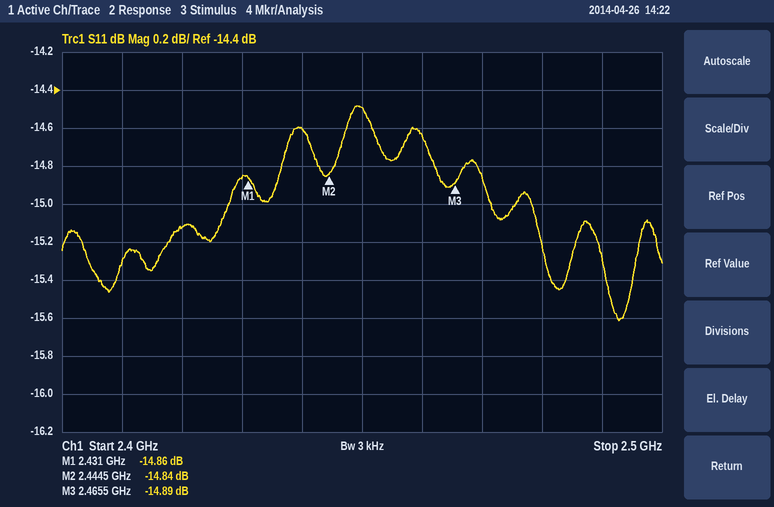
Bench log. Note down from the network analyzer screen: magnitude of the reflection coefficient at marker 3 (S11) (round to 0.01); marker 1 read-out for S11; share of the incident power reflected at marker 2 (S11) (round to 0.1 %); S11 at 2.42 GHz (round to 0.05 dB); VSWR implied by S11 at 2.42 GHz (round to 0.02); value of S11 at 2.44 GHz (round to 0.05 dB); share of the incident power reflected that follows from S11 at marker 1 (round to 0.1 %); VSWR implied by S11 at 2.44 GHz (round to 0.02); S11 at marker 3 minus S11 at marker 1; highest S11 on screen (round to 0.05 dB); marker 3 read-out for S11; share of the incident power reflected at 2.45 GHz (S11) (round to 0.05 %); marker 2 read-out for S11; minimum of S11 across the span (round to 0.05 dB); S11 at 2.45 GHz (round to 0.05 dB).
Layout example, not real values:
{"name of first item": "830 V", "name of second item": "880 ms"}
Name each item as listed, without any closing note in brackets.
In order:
{"magnitude of the reflection coefficient at marker 3 (S11)": "0.18", "marker 1 read-out for S11": "-14.86 dB", "share of the incident power reflected at marker 2 (S11)": "3.3 %", "S11 at 2.42 GHz": "-15.10 dB", "VSWR implied by S11 at 2.42 GHz": "1.42", "value of S11 at 2.44 GHz": "-14.60 dB", "share of the incident power reflected that follows from S11 at marker 1": "3.3 %", "VSWR implied by S11 at 2.44 GHz": "1.46", "S11 at marker 3 minus S11 at marker 1": "-0.03 dB", "highest S11 on screen": "-14.50 dB", "marker 3 read-out for S11": "-14.89 dB", "share of the incident power reflected at 2.45 GHz (S11)": "3.55 %", "marker 2 read-out for S11": "-14.84 dB", "minimum of S11 across the span": "-15.60 dB", "S11 at 2.45 GHz": "-14.50 dB"}
